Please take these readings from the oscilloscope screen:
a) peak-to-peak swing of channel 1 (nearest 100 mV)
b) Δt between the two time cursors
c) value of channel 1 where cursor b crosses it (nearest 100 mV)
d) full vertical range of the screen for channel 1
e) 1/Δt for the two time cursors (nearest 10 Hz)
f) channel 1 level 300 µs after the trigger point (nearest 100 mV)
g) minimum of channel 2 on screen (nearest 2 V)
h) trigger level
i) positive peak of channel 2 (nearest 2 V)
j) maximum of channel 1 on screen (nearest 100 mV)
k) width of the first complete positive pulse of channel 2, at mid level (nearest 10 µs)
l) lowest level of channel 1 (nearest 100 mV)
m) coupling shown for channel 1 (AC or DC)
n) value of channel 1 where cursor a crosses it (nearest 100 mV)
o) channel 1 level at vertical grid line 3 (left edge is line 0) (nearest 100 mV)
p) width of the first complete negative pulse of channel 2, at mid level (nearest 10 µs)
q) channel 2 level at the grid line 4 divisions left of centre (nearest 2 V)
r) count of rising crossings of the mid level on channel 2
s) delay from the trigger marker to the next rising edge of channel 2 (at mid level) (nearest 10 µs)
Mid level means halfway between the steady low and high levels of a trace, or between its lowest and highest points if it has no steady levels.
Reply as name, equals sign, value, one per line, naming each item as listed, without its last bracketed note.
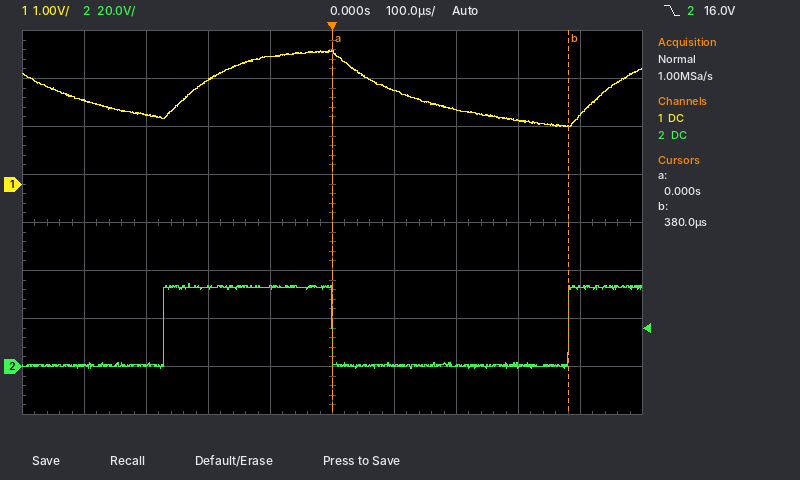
peak-to-peak swing of channel 1 = 1.6 V
Δt between the two time cursors = 380 µs
value of channel 1 where cursor b crosses it = 1.2 V
full vertical range of the screen for channel 1 = 8 V
1/Δt for the two time cursors = 2.63 kHz
channel 1 level 300 µs after the trigger point = 1.3 V
minimum of channel 2 on screen = 0 V
trigger level = 16.0 V
positive peak of channel 2 = 34 V
maximum of channel 1 on screen = 2.8 V
width of the first complete positive pulse of channel 2, at mid level = 270 µs
lowest level of channel 1 = 1.2 V
coupling shown for channel 1 = DC
value of channel 1 where cursor a crosses it = 2.7 V
channel 1 level at vertical grid line 3 (left edge is line 0) = 2.2 V
width of the first complete negative pulse of channel 2, at mid level = 380 µs
channel 2 level at the grid line 4 divisions left of centre = 0 V
count of rising crossings of the mid level on channel 2 = 2
delay from the trigger marker to the next rising edge of channel 2 (at mid level) = 380 µs
